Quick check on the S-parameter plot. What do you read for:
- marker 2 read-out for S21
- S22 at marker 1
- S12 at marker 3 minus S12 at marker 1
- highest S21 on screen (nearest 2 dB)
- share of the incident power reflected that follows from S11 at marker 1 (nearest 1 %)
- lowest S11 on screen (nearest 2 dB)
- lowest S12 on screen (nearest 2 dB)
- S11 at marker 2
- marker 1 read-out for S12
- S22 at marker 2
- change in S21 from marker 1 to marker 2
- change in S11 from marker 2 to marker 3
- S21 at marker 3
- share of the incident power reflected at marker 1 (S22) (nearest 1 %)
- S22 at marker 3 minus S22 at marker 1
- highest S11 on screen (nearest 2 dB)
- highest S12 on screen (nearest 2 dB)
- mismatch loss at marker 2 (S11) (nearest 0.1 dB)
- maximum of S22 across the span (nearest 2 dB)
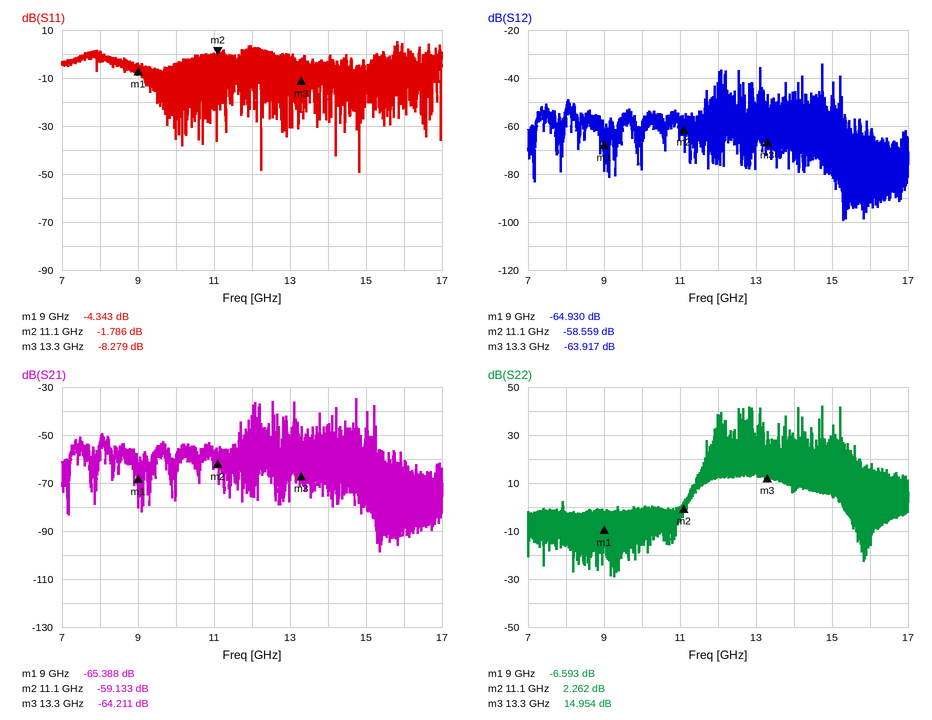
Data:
-59.133 dB
-6.593 dB
1.013 dB
-34 dB
37 %
-50 dB
-100 dB
-1.786 dB
-64.930 dB
2.262 dB
6.255 dB
-6.493 dB
-64.211 dB
22 %
21.547 dB
6 dB
-34 dB
4.7 dB
42 dB
